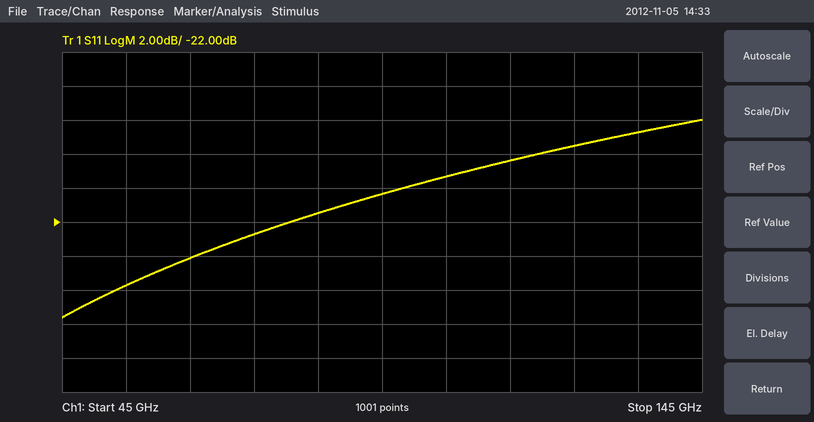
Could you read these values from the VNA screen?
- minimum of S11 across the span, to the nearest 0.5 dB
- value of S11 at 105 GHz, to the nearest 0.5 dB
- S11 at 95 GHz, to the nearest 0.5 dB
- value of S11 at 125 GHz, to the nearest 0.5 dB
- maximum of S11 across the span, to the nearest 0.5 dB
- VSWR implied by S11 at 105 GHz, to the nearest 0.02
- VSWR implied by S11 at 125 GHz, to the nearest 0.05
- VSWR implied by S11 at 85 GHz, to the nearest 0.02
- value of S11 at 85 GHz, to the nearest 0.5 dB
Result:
-27.5 dB
-19.5 dB
-20.5 dB
-17.5 dB
-16.0 dB
1.24
1.30
1.18
-21.5 dB
